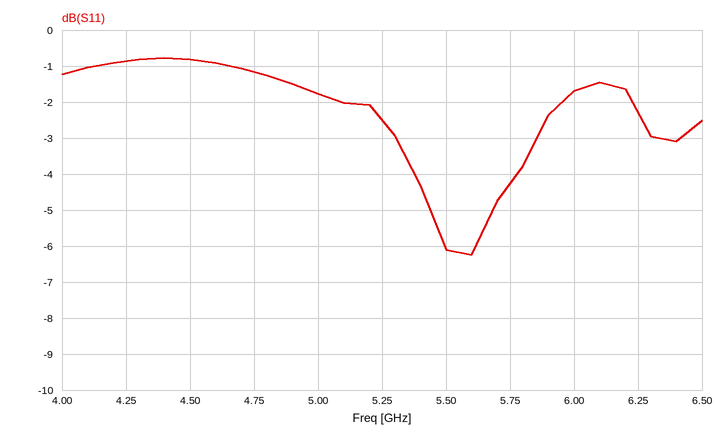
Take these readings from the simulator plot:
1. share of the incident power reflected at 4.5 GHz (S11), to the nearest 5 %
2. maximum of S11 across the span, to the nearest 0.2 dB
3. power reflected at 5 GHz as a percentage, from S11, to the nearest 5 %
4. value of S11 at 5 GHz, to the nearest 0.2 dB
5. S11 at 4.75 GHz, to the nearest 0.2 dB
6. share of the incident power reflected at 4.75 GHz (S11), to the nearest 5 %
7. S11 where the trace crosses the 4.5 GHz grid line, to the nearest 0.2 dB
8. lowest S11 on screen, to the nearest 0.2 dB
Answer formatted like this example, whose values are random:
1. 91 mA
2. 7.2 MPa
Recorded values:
1. 85 %
2. -0.8 dB
3. 65 %
4. -1.8 dB
5. -1.2 dB
6. 75 %
7. -0.8 dB
8. -6.2 dB
